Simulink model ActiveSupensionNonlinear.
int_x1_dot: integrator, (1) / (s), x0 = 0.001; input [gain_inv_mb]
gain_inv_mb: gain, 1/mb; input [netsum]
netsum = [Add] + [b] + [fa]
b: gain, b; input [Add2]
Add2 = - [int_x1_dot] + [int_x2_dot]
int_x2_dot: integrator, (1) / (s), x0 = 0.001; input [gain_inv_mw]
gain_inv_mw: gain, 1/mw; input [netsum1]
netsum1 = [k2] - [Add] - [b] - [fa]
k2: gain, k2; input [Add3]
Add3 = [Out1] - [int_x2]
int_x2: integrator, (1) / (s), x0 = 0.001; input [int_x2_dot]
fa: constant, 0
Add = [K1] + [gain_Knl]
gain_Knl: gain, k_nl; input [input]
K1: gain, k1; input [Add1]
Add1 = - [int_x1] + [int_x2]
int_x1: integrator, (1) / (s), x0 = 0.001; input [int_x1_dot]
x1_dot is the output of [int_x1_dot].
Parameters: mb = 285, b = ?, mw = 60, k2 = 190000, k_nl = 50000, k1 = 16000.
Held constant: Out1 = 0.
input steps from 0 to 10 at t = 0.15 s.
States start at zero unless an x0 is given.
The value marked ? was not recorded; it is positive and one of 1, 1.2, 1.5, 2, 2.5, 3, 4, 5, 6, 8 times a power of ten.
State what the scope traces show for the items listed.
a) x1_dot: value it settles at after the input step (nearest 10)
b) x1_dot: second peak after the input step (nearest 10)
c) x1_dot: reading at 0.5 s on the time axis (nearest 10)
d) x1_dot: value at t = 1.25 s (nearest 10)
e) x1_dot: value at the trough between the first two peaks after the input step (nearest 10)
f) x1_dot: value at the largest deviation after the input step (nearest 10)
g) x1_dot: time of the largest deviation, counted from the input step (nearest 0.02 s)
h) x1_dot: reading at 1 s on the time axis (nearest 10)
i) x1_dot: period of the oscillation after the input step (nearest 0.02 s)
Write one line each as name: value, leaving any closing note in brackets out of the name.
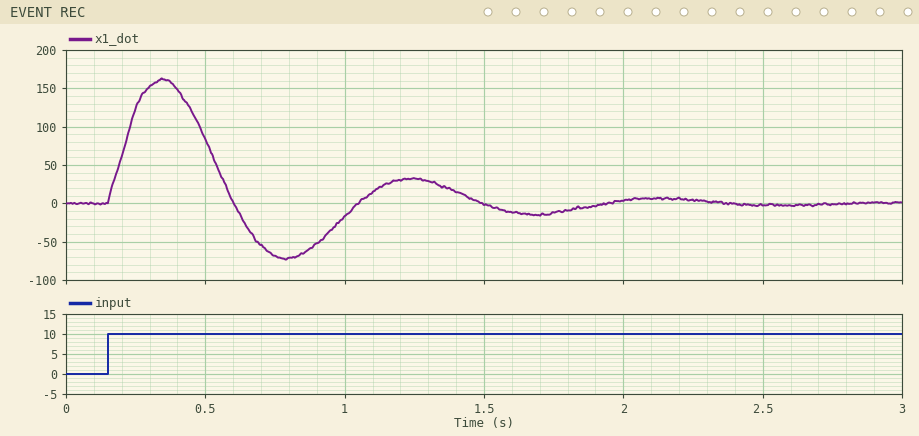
x1_dot: value it settles at after the input step: 0
x1_dot: second peak after the input step: 30
x1_dot: reading at 0.5 s on the time axis: 80
x1_dot: value at t = 1.25 s: 30
x1_dot: value at the trough between the first two peaks after the input step: -70
x1_dot: value at the largest deviation after the input step: 160
x1_dot: time of the largest deviation, counted from the input step: 0.20 s
x1_dot: reading at 1 s on the time axis: -20
x1_dot: period of the oscillation after the input step: 0.88 s
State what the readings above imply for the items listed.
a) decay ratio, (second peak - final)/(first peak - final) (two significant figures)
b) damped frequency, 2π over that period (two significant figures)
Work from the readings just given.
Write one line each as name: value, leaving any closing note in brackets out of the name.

decay ratio, (second peak - final)/(first peak - final): 0.19
damped frequency, 2π over that period: 7.1 rad/s
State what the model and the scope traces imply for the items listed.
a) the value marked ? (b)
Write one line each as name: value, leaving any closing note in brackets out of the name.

the value marked ?: 1200
